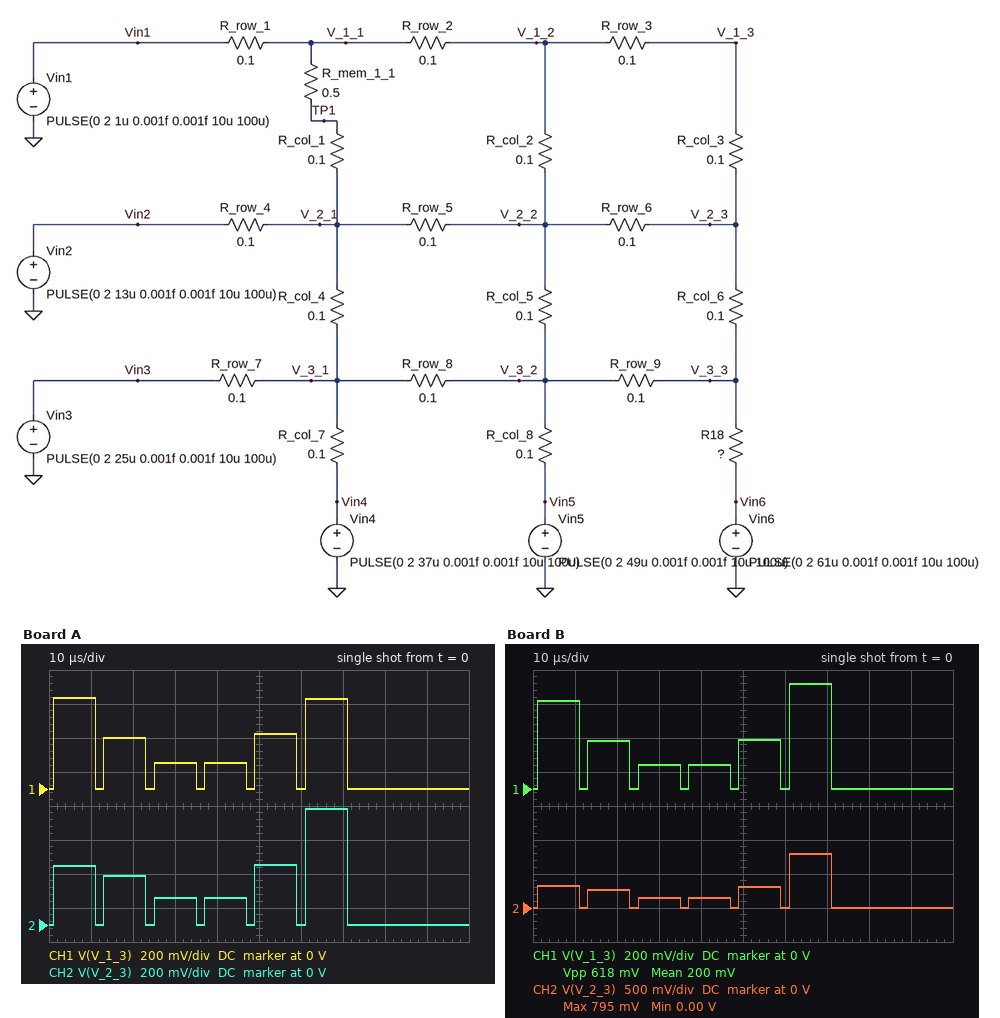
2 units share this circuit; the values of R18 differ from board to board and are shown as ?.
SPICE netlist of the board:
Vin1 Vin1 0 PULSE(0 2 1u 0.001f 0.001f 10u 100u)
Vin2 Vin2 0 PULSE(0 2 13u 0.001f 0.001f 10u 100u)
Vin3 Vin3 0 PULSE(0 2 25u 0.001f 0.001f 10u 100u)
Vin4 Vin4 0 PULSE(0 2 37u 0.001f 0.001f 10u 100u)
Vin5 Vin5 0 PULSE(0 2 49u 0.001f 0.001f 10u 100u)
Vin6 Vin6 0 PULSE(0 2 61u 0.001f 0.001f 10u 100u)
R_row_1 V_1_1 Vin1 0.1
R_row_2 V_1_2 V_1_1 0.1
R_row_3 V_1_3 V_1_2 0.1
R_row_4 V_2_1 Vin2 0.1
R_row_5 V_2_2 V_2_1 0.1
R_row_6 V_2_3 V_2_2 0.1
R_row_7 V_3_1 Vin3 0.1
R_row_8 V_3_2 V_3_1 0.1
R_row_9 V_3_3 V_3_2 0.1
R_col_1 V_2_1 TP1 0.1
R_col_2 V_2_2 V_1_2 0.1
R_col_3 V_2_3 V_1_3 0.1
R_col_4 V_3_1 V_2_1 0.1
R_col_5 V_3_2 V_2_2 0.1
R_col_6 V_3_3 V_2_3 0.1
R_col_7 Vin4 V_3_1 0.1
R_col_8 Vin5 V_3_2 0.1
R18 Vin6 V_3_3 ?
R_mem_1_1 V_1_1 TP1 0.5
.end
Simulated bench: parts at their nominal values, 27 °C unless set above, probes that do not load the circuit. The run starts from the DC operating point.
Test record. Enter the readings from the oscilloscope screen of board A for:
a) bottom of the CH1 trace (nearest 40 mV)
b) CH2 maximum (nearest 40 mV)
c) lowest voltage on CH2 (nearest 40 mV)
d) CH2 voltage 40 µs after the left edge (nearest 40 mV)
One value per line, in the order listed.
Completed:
0 V
680 mV
0 V
160 mV
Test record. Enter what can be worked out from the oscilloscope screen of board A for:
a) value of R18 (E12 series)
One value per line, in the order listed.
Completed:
0.082 Ω
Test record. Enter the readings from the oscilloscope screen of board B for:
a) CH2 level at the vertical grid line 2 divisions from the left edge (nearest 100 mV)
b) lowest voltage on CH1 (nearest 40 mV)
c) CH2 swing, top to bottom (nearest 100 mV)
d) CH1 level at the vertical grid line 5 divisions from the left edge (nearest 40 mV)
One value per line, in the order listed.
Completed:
300 mV
0 V
800 mV
280 mV
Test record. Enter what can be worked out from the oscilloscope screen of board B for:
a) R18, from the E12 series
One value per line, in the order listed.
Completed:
0.056 Ω
